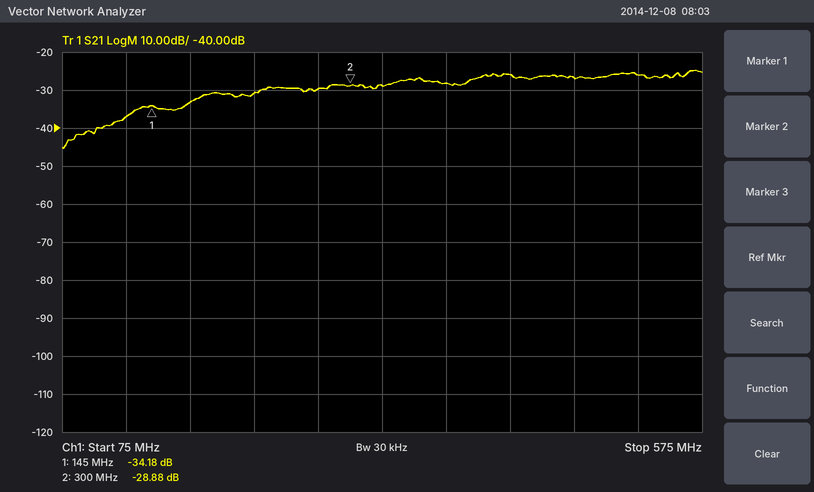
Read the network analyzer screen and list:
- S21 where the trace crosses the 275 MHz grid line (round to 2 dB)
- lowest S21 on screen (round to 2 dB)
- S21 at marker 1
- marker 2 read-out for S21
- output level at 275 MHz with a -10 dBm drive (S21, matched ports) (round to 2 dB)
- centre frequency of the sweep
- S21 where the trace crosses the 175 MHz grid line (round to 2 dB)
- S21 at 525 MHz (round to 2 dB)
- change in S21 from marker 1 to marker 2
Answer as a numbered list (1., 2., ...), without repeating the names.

1. -30 dB
2. -46 dB
3. -34.18 dB
4. -28.88 dB
5. -40 dBm
6. 325 MHz
7. -34 dB
8. -26 dB
9. 5.30 dB
